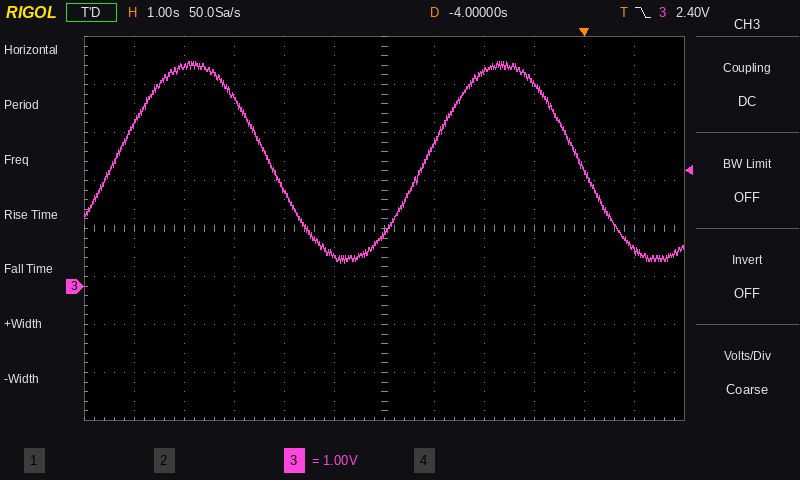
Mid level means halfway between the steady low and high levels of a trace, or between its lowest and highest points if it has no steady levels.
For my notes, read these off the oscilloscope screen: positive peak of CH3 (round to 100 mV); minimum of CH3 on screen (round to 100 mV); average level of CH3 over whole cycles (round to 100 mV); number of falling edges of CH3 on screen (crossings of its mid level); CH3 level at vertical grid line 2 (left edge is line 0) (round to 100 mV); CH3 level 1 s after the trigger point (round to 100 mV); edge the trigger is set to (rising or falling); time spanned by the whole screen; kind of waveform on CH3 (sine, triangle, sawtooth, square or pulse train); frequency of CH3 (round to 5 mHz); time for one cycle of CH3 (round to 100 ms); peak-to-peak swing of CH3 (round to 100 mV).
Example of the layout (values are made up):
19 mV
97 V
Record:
4.7 V
500 mV
2.6 V
2
4.6 V
700 mV
falling
12 s
sine
160 mHz
6.2 s
4.2 V
